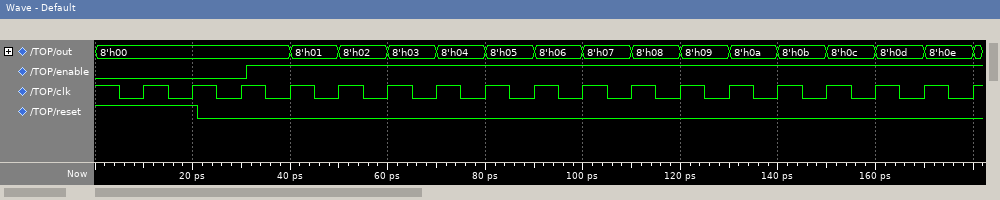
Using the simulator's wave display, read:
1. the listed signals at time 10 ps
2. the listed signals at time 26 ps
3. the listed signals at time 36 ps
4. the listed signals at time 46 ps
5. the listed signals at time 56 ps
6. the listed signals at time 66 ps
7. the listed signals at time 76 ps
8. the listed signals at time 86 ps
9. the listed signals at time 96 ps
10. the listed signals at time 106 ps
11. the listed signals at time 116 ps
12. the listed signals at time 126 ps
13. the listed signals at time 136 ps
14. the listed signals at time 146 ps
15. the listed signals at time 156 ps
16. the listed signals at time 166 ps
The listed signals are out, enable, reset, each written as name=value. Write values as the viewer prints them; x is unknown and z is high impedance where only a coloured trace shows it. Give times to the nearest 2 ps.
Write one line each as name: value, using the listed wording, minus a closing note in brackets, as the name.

the listed signals at time 10 ps: out=8'h00, enable=0, reset=1
the listed signals at time 26 ps: out=8'h00, enable=0, reset=0
the listed signals at time 36 ps: out=8'h00, enable=1, reset=0
the listed signals at time 46 ps: out=8'h01, enable=1, reset=0
the listed signals at time 56 ps: out=8'h02, enable=1, reset=0
the listed signals at time 66 ps: out=8'h03, enable=1, reset=0
the listed signals at time 76 ps: out=8'h04, enable=1, reset=0
the listed signals at time 86 ps: out=8'h05, enable=1, reset=0
the listed signals at time 96 ps: out=8'h06, enable=1, reset=0
the listed signals at time 106 ps: out=8'h07, enable=1, reset=0
the listed signals at time 116 ps: out=8'h08, enable=1, reset=0
the listed signals at time 126 ps: out=8'h09, enable=1, reset=0
the listed signals at time 136 ps: out=8'h0a, enable=1, reset=0
the listed signals at time 146 ps: out=8'h0b, enable=1, reset=0
the listed signals at time 156 ps: out=8'h0c, enable=1, reset=0
the listed signals at time 166 ps: out=8'h0d, enable=1, reset=0
